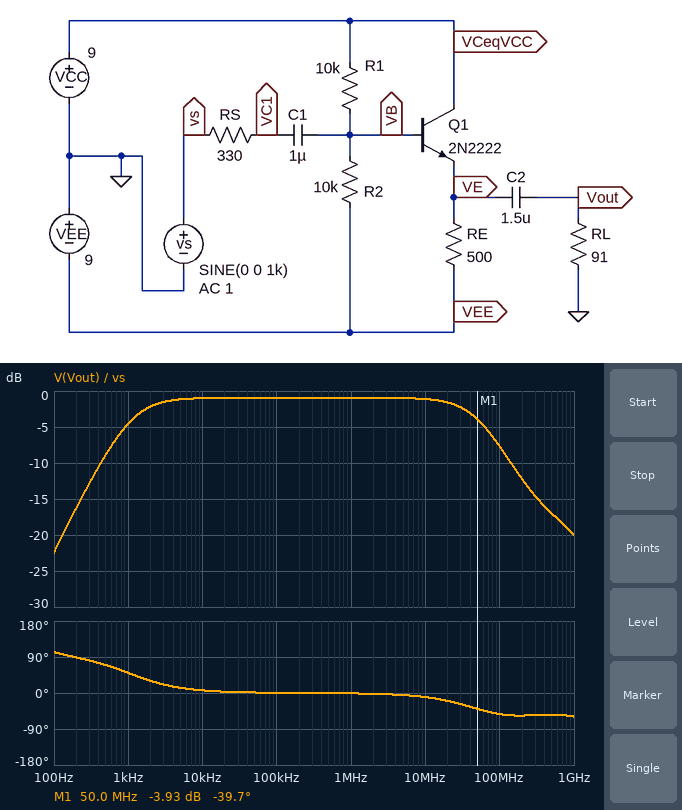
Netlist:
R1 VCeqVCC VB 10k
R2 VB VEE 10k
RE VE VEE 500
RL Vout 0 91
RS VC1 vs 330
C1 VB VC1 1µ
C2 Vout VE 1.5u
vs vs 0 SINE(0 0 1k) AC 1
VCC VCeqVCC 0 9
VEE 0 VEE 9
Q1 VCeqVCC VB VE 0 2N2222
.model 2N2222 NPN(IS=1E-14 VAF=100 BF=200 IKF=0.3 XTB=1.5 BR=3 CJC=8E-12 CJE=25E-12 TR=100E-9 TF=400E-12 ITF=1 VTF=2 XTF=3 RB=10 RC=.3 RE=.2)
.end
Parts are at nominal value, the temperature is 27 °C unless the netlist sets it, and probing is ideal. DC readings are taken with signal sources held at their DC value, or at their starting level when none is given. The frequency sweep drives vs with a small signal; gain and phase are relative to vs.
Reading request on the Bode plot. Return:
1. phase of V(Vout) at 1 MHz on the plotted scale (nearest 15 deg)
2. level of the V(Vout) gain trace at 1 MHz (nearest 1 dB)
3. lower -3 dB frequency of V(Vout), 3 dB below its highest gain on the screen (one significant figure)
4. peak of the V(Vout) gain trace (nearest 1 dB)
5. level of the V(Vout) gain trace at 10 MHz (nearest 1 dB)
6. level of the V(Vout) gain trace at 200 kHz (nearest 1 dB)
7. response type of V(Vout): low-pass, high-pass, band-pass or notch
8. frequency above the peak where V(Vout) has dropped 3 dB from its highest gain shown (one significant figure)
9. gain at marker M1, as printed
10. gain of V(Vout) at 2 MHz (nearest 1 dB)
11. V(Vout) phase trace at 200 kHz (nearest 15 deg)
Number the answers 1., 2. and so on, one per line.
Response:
1. 0 deg
2. -1 dB
3. 1 kHz
4. -1 dB
5. -1 dB
6. -1 dB
7. band-pass
8. 50 MHz
9. -3.93 dB
10. -1 dB
11. 0 deg
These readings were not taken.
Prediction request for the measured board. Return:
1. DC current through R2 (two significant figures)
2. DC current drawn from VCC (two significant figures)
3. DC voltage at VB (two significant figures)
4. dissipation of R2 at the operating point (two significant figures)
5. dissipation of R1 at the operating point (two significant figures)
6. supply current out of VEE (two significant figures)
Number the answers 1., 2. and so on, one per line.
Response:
1. 860 µA
2. 17 mA
3. -380 mV
4. 7.4 mW
5. 8.8 mW
6. 17 mA
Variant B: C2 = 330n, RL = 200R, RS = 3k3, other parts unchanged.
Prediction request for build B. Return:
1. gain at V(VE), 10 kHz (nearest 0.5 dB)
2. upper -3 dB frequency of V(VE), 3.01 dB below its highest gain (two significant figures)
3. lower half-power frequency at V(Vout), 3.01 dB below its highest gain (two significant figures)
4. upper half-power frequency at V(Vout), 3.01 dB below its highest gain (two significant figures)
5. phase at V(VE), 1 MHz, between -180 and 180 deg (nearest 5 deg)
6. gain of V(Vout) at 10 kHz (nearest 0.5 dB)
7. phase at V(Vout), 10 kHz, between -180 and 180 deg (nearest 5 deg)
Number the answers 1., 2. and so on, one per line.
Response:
1. -5.0 dB
2. 11 MHz
3. 2.3 kHz
4. 13 MHz
5. -5 deg
6. -5.5 dB
7. 15 deg
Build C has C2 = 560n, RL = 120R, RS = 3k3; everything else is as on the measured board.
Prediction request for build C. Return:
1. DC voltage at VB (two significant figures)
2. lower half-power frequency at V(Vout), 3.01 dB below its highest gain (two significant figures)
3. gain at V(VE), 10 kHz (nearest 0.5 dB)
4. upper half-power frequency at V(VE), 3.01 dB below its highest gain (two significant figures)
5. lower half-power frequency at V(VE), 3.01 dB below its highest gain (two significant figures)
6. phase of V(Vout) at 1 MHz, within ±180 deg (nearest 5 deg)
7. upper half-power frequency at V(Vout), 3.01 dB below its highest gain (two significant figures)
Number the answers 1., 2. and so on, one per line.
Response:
1. -380 mV
2. 2.2 kHz
3. -5.5 dB
4. 8.7 MHz
5. 20 Hz
6. -5 deg
7. 11 MHz
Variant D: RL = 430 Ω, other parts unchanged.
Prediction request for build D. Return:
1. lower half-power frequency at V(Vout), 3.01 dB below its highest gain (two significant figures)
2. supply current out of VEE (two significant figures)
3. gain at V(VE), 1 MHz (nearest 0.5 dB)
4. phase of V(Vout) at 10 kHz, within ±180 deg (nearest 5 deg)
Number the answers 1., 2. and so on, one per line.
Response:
1. 250 Hz
2. 17 mA
3. -0.5 dB
4. 0 deg
